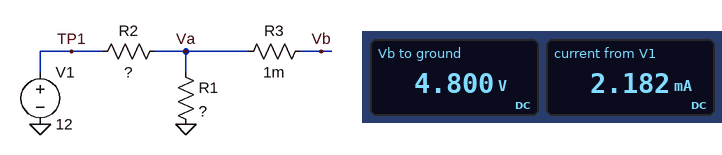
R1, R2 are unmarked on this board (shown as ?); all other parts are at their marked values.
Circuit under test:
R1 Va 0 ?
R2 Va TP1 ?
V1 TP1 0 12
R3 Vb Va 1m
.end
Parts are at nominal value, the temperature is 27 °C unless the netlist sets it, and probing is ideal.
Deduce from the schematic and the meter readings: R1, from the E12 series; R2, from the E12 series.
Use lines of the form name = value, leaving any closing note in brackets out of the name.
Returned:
R1, from the E12 series = 2.2 kΩ
R2, from the E12 series = 3.3 kΩ
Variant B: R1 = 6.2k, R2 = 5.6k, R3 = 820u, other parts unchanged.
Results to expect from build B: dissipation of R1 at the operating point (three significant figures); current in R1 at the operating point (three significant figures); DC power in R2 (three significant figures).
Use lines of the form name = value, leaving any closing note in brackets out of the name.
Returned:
dissipation of R1 at the operating point = 6.41 mW
current in R1 at the operating point = 1.02 mA
DC power in R2 = 5.79 mW
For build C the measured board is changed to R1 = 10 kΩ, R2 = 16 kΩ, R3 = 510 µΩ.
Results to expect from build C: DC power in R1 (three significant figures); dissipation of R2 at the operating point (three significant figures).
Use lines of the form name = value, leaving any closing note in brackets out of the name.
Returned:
DC power in R1 = 2.13 mW
dissipation of R2 at the operating point = 3.41 mW
